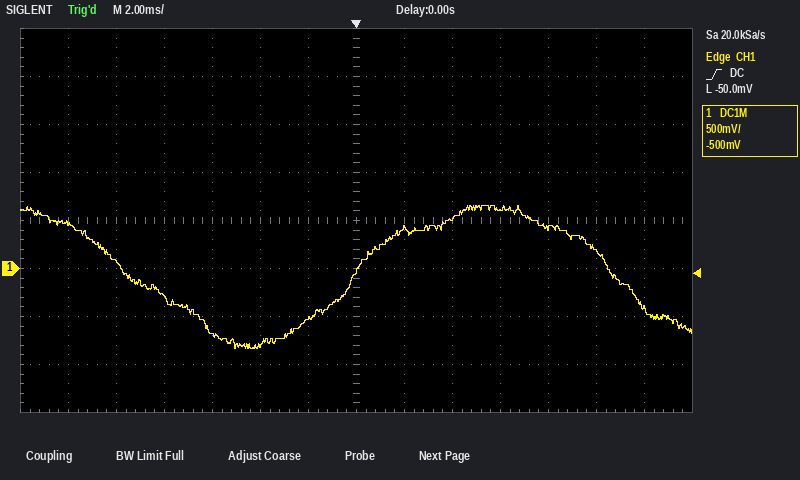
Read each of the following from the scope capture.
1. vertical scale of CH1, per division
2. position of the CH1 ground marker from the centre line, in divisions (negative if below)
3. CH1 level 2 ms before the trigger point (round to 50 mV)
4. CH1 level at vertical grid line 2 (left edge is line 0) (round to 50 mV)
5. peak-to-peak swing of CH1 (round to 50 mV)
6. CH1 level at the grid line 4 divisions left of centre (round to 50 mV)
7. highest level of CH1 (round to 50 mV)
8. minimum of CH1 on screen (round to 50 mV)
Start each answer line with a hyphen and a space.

- 500 mV
- -1.0 div
- -500 mV
- 50 mV
- 1.50 V
- -300 mV
- 650 mV
- -850 mV
